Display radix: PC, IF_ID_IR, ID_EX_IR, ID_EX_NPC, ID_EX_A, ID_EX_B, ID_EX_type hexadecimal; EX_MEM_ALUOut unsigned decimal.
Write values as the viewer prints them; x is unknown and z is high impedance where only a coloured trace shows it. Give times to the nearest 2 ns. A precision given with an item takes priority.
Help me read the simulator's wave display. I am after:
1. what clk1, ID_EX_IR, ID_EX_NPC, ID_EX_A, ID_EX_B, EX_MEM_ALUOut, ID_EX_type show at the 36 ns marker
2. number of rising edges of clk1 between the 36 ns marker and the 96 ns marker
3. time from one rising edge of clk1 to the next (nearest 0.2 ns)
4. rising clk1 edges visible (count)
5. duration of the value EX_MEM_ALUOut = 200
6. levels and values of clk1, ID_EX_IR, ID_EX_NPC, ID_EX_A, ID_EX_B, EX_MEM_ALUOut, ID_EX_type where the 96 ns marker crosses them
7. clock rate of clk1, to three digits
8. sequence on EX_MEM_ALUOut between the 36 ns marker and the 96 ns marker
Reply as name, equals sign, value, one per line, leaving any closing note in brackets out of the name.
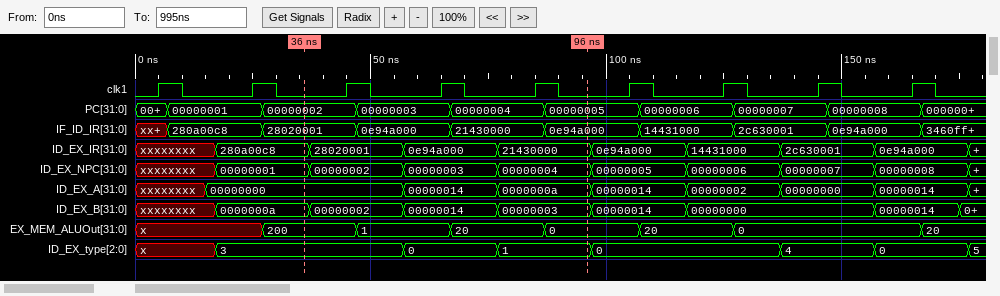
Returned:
what clk1, ID_EX_IR, ID_EX_NPC, ID_EX_A, ID_EX_B, EX_MEM_ALUOut, ID_EX_type show at the 36 ns marker = clk1=0, ID_EX_IR=280a00c8, ID_EX_NPC=00000001, ID_EX_A=00000000, ID_EX_B=0000000a, EX_MEM_ALUOut=200, ID_EX_type=3
number of rising edges of clk1 between the 36 ns marker and the 96 ns marker = 3
time from one rising edge of clk1 to the next = 20 ns
rising clk1 edges visible = 9
duration of the value EX_MEM_ALUOut = 200 = 20 ns
levels and values of clk1, ID_EX_IR, ID_EX_NPC, ID_EX_A, ID_EX_B, EX_MEM_ALUOut, ID_EX_type where the 96 ns marker crosses them = clk1=0, ID_EX_IR=21430000, ID_EX_NPC=00000004, ID_EX_A=0000000a, ID_EX_B=00000003, EX_MEM_ALUOut=0, ID_EX_type=1
clock rate of clk1, to three digits = 50.0 MHz
sequence on EX_MEM_ALUOut between the 36 ns marker and the 96 ns marker = 200, 1, 20, 0
